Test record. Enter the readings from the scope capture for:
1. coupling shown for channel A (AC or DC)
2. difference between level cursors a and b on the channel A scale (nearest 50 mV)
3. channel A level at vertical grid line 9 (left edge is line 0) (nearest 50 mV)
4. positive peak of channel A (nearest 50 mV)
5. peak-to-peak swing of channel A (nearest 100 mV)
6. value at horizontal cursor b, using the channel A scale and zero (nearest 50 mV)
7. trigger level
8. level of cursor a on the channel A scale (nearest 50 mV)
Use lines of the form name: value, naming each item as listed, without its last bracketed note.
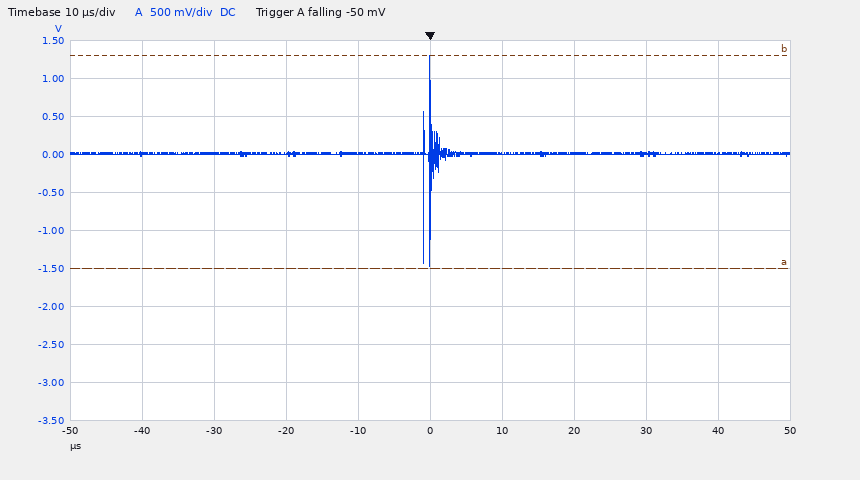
coupling shown for channel A: DC
difference between level cursors a and b on the channel A scale: 2.80 V
channel A level at vertical grid line 9 (left edge is line 0): 0 mV
positive peak of channel A: 1.30 V
peak-to-peak swing of channel A: 2.80 V
value at horizontal cursor b, using the channel A scale and zero: 1.30 V
trigger level: -50 mV
level of cursor a on the channel A scale: -1.50 V
